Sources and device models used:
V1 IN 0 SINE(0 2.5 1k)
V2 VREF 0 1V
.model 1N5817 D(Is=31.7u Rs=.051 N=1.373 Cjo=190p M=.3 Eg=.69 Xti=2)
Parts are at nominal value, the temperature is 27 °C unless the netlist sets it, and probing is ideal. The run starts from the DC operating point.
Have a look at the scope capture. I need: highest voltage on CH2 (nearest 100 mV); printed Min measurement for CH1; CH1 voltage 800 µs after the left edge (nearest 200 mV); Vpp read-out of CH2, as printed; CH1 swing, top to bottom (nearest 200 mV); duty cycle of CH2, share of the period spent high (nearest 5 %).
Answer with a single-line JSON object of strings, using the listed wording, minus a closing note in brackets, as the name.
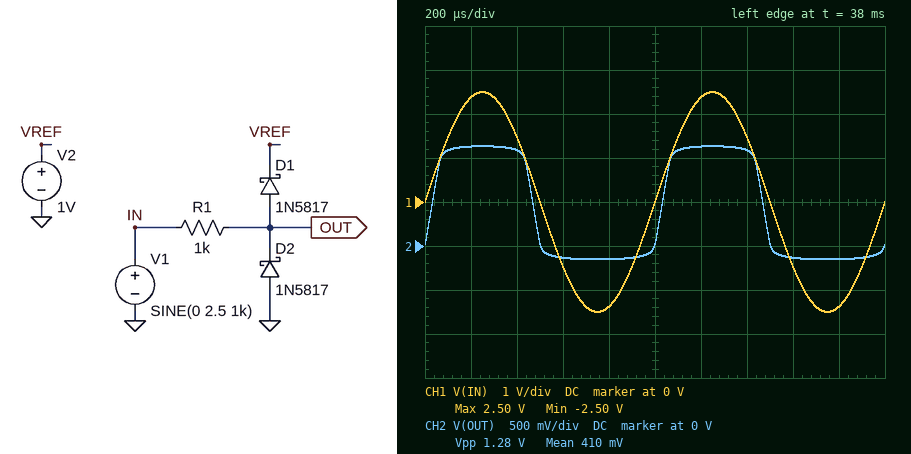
{"highest voltage on CH2": "1.1 V", "printed Min measurement for CH1": "-2.50 V", "CH1 voltage 800 µs after the left edge": "-2.4 V", "Vpp read-out of CH2, as printed": "1.28 V", "CH1 swing, top to bottom": "5.0 V", "duty cycle of CH2, share of the period spent high": "45 %"}
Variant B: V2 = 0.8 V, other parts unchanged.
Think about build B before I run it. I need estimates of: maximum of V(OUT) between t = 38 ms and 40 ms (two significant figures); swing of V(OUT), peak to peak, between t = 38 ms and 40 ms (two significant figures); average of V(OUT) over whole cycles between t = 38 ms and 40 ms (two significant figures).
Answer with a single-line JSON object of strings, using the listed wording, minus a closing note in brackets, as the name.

{"maximum of V(OUT) between t = 38 ms and 40 ms": "940 mV", "swing of V(OUT), peak to peak, between t = 38 ms and 40 ms": "1.1 V", "average of V(OUT) over whole cycles between t = 38 ms and 40 ms": "340 mV"}
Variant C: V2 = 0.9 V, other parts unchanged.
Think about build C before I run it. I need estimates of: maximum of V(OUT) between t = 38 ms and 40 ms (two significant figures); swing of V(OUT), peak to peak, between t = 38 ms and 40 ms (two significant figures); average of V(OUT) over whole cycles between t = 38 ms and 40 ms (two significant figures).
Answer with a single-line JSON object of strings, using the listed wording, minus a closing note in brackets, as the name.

{"maximum of V(OUT) between t = 38 ms and 40 ms": "1.0 V", "swing of V(OUT), peak to peak, between t = 38 ms and 40 ms": "1.2 V", "average of V(OUT) over whole cycles between t = 38 ms and 40 ms": "380 mV"}
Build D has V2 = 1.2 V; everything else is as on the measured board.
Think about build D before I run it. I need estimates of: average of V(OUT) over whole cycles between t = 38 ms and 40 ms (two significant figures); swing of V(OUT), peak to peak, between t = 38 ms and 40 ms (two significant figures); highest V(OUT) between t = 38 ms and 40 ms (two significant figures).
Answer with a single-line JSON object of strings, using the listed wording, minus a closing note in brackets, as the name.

{"average of V(OUT) over whole cycles between t = 38 ms and 40 ms": "480 mV", "swing of V(OUT), peak to peak, between t = 38 ms and 40 ms": "1.5 V", "highest V(OUT) between t = 38 ms and 40 ms": "1.3 V"}
